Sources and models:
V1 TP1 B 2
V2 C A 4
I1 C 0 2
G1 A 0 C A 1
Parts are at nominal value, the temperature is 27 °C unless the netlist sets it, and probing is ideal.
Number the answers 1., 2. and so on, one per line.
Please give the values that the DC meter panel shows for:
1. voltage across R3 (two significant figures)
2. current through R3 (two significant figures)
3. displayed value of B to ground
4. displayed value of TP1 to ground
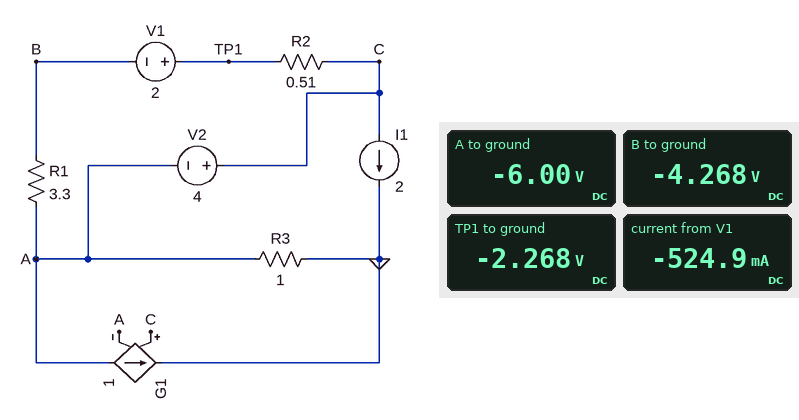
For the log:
1. 6.0 V
2. 6.0 A
3. -4.268 V
4. -2.268 V
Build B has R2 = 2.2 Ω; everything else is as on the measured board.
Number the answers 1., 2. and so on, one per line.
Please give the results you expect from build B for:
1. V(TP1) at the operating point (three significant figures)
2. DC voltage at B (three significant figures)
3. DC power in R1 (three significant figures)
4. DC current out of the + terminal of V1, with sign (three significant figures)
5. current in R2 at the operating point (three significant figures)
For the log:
1. -2.80 V
2. -4.80 V
3. 436 mW
4. -364 mA
5. 364 mA
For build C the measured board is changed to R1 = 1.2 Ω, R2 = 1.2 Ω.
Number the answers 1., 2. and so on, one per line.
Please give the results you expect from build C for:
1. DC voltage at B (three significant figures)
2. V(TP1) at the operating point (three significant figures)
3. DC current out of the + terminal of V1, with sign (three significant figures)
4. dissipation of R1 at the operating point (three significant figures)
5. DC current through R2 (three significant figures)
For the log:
1. -5.00 V
2. -3.00 V
3. -833 mA
4. 833 mW
5. 833 mA
